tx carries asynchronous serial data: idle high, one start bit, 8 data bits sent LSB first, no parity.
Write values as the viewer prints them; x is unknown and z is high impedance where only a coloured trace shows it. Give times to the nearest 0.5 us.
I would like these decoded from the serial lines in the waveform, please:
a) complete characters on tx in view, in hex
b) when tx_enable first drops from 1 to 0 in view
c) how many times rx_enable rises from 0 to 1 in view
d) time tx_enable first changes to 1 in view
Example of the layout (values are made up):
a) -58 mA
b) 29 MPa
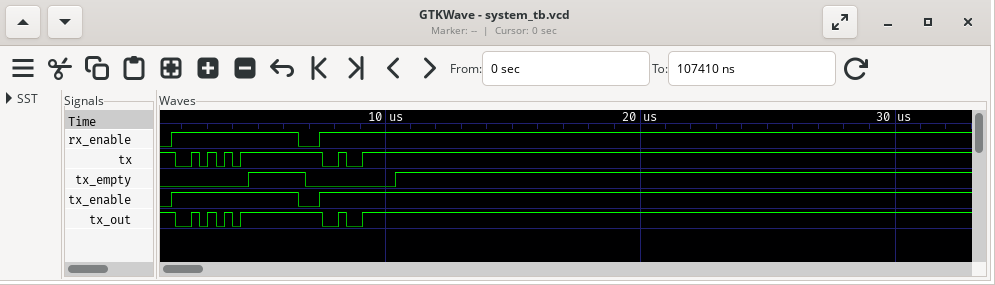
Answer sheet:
a) AA, F2
b) 6.5 us
c) 2
d) 1.5 us
